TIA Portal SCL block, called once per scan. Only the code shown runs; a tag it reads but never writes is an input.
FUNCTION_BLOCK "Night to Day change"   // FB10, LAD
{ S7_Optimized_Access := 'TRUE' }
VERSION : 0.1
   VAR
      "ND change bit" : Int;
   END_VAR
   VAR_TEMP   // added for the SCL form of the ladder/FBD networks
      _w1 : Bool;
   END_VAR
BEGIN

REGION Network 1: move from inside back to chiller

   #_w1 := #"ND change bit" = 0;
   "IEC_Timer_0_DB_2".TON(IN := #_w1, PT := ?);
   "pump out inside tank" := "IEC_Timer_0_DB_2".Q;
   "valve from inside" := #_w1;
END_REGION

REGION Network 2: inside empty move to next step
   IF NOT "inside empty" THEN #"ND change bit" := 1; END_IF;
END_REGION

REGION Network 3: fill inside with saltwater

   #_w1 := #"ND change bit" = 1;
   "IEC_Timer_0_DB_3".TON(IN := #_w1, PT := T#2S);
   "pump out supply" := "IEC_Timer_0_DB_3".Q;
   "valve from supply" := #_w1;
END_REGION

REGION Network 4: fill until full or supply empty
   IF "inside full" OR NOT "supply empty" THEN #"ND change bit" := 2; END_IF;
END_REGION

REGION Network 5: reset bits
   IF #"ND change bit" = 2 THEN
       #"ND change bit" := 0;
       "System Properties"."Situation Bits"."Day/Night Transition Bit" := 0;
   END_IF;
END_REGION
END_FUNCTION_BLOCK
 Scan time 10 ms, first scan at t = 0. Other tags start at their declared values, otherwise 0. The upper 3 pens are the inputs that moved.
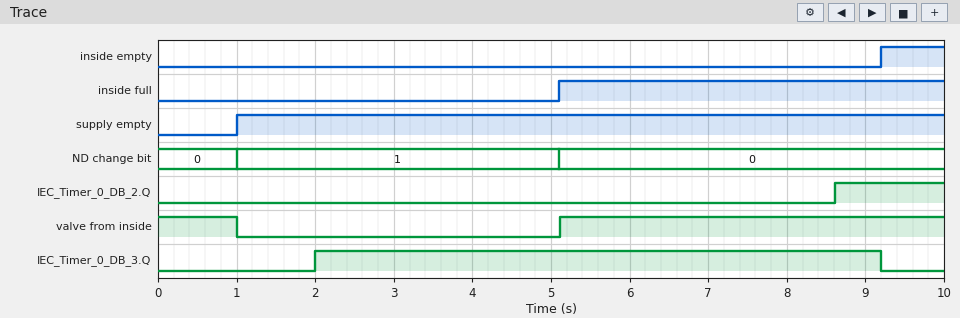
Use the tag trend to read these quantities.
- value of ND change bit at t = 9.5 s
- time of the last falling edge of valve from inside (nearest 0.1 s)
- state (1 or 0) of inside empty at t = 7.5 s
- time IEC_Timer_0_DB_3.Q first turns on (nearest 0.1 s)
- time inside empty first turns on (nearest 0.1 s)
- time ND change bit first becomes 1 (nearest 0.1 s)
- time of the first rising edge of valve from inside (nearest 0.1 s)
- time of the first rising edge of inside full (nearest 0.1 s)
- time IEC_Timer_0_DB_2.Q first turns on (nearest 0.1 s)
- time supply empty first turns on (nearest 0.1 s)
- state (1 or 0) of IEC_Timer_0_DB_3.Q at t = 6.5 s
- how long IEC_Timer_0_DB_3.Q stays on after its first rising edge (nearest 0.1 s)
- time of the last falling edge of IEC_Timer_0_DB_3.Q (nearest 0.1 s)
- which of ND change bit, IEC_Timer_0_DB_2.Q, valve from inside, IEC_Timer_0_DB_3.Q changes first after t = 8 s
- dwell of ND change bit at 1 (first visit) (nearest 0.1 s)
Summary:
0
1.0 s
0
2.0 s
9.2 s
1.0 s
5.1 s
5.1 s
8.6 s
1.0 s
1
7.2 s
9.2 s
IEC_Timer_0_DB_2.Q
4.1 s
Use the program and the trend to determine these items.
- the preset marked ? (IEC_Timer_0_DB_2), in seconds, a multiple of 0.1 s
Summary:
3.5 s
